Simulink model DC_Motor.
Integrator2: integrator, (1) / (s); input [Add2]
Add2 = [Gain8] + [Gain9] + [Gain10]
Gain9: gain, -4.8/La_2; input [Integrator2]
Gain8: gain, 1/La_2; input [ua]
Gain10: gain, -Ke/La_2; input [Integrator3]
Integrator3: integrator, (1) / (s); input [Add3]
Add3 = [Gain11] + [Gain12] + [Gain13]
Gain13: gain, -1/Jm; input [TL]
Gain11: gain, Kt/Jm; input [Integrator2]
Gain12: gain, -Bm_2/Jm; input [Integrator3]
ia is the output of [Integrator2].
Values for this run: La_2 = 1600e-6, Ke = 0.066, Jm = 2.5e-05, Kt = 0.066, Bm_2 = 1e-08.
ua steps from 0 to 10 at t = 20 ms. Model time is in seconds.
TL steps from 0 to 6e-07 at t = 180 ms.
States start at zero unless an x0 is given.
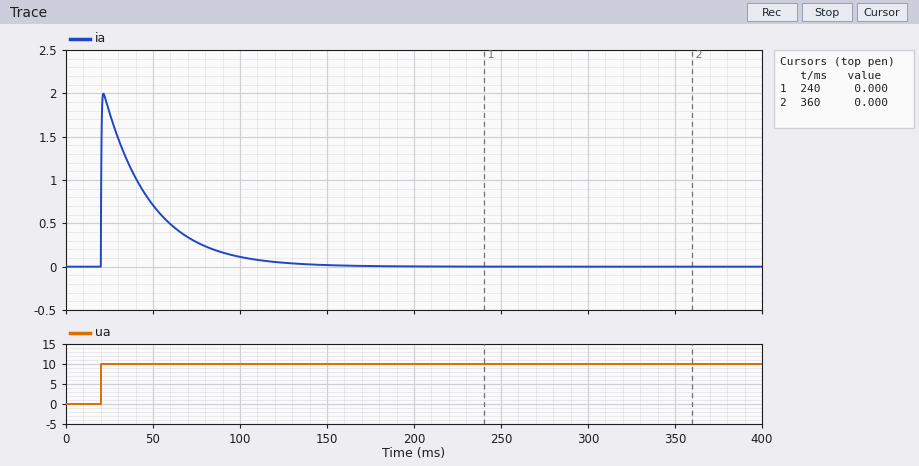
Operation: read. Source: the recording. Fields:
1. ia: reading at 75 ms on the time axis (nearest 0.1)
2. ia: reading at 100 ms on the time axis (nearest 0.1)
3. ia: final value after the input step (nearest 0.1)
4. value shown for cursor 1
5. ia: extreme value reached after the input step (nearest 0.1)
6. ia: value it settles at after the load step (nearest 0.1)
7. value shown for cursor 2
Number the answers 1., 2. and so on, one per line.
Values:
1. 0.3
2. 0.1
3. 0.0
4. 0.000
5. 2.0
6. 0.0
7. 0.000
